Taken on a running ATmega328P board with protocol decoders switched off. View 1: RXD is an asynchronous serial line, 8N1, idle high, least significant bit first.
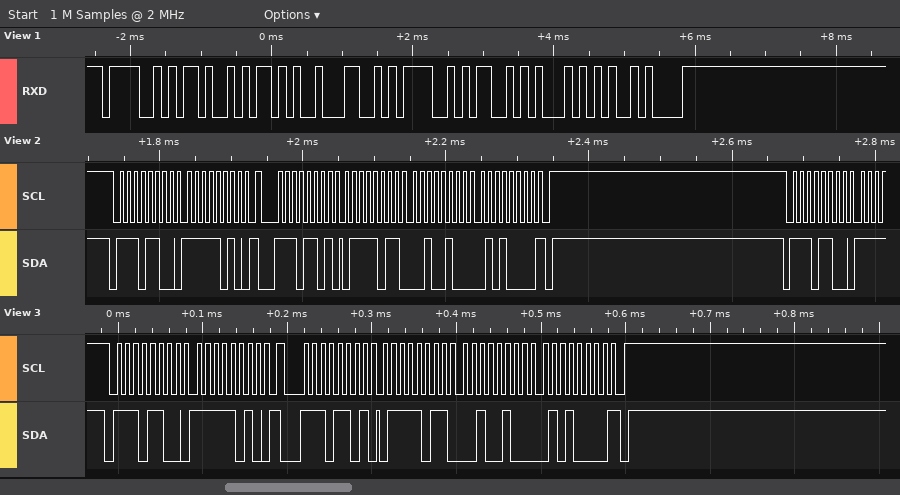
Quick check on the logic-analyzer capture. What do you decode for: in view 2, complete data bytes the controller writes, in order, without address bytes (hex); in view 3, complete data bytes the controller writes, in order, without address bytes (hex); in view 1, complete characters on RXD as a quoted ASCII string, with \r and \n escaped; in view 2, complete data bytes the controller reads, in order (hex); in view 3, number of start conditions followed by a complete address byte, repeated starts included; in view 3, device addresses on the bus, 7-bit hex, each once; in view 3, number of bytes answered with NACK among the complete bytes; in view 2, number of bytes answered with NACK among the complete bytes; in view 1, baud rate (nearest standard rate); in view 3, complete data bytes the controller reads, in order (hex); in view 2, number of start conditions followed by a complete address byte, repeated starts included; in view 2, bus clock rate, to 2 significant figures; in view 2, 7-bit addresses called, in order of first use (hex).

FA
FA
"OK+LOST\n"
7B 24 50
2
0x76
1
1
9600 baud
7B 24 50
3
100 kHz
0x76
